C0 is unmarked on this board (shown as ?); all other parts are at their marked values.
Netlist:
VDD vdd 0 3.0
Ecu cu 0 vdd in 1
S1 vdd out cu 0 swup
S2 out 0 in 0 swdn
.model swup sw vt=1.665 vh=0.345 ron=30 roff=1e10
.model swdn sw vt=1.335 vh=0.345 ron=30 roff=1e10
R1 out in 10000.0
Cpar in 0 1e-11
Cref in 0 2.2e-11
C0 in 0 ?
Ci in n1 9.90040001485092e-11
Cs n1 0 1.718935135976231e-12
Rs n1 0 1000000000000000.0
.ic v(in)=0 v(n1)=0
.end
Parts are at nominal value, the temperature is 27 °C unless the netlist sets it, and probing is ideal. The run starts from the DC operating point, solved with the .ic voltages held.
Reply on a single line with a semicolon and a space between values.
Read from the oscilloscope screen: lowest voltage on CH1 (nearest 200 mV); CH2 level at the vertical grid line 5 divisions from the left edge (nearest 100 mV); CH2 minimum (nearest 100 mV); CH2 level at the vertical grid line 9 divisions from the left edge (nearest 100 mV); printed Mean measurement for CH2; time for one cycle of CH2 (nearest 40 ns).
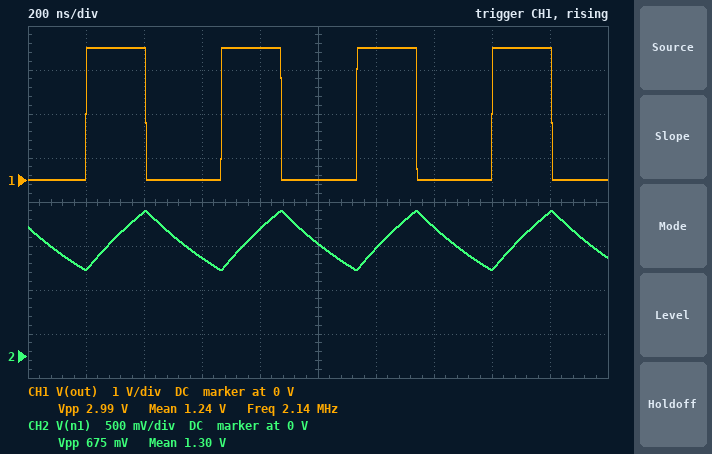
0 V; 1.3 V; 1.0 V; 1.6 V; 1.30 V; 480 ns
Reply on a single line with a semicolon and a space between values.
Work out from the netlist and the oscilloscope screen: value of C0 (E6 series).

15 pF
